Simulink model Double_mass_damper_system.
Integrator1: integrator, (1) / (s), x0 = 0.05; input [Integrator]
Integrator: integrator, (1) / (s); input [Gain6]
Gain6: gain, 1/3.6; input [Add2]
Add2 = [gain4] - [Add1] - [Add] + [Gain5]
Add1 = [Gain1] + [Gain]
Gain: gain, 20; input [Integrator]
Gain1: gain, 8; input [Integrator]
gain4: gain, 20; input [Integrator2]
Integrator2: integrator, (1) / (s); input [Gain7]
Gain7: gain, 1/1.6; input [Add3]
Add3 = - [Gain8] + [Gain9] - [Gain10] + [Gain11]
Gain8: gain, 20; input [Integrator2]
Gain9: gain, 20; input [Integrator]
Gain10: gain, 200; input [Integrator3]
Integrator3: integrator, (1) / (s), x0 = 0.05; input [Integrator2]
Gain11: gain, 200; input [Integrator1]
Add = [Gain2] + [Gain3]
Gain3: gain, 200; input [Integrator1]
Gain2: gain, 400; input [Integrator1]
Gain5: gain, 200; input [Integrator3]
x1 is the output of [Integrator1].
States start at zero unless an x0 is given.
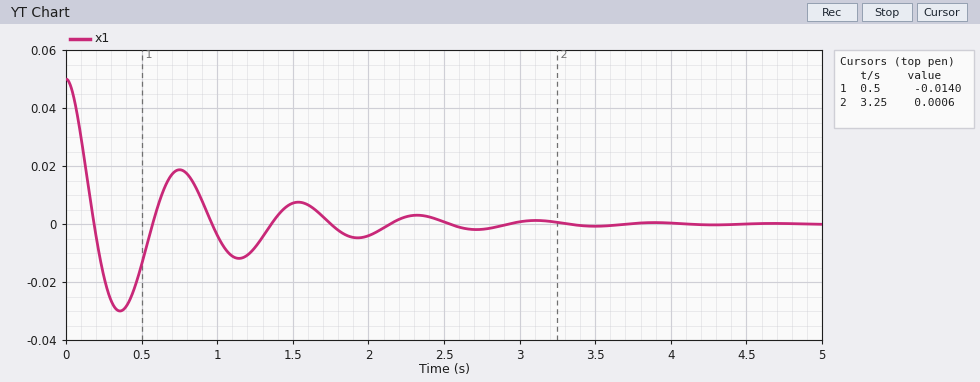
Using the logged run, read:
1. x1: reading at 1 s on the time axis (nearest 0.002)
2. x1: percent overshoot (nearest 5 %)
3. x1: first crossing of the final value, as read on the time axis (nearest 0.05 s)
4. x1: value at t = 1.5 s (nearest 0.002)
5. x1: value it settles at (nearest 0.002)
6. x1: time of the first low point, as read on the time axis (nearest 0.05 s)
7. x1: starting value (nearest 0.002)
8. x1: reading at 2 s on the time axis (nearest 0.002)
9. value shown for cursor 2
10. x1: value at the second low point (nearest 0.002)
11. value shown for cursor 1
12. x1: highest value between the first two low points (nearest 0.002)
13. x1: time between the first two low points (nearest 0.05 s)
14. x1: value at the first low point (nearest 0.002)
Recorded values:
-0.004
60 %
0.20 s
0.008
0.000
0.35 s
0.050
-0.004
0.0006
-0.012
-0.0140
0.018
0.80 s
-0.030
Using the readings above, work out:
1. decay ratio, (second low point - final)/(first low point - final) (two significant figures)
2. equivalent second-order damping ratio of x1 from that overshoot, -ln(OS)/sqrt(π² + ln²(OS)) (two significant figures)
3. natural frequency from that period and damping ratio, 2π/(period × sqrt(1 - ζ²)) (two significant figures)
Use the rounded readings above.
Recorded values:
0.40
0.16
8.0 rad/s
